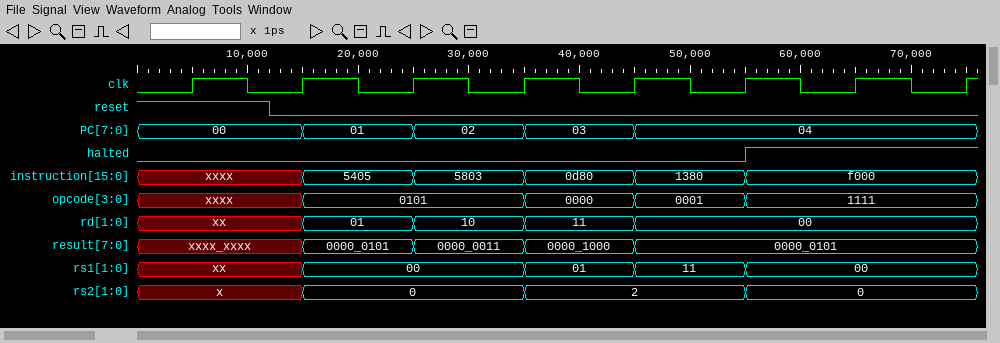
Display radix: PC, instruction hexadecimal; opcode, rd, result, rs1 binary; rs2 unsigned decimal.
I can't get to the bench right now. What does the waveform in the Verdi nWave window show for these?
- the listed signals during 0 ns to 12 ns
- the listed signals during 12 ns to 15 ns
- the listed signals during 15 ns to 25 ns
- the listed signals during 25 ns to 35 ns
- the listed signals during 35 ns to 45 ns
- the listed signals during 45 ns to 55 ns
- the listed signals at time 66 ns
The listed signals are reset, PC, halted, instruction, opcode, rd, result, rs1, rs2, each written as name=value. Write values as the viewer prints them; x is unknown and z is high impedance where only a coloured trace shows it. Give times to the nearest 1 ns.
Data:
reset=1, PC=00, halted=0, instruction=xxxx, opcode=xxxx, rd=xx, result=xxxx_xxxx, rs1=xx, rs2=x
reset=0, PC=00, halted=0, instruction=xxxx, opcode=xxxx, rd=xx, result=xxxx_xxxx, rs1=xx, rs2=x
reset=0, PC=01, halted=0, instruction=5405, opcode=0101, rd=01, result=0000_0101, rs1=00, rs2=0
reset=0, PC=02, halted=0, instruction=5803, opcode=0101, rd=10, result=0000_0011, rs1=00, rs2=0
reset=0, PC=03, halted=0, instruction=0d80, opcode=0000, rd=11, result=0000_1000, rs1=01, rs2=2
reset=0, PC=04, halted=0, instruction=1380, opcode=0001, rd=00, result=0000_0101, rs1=11, rs2=2
reset=0, PC=04, halted=1, instruction=f000, opcode=1111, rd=00, result=0000_0101, rs1=00, rs2=0
